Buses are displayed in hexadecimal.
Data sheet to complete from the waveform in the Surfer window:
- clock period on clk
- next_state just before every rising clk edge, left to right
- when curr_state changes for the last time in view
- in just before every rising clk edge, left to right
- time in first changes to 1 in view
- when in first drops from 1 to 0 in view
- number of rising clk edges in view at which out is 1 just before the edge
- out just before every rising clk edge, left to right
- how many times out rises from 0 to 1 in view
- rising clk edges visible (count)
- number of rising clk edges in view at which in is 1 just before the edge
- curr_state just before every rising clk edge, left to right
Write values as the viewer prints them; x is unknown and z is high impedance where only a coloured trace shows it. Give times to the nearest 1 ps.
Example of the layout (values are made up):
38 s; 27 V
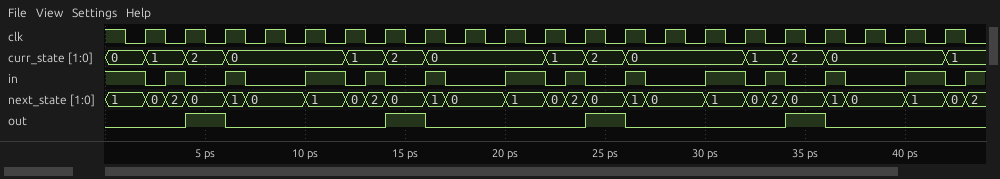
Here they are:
2 ps; 1, 2, 0, 0, 0, 1, 2, 0, 0, 0, 1, 2, 0, 0, 0, 1, 2, 0, 0, 0, 1; 42 ps; 1 1 0 0 0 1 1 0 0 0 1 1 0 0 0 1 1 0 0 0 1; 3 ps; 2 ps; 4; 0 0 1 0 0 0 0 1 0 0 0 0 1 0 0 0 0 1 0 0 0; 4; 21; 9; 0, 1, 2, 0, 0, 0, 1, 2, 0, 0, 0, 1, 2, 0, 0, 0, 1, 2, 0, 0, 0
